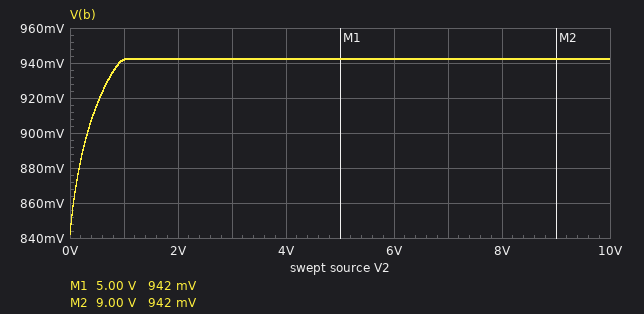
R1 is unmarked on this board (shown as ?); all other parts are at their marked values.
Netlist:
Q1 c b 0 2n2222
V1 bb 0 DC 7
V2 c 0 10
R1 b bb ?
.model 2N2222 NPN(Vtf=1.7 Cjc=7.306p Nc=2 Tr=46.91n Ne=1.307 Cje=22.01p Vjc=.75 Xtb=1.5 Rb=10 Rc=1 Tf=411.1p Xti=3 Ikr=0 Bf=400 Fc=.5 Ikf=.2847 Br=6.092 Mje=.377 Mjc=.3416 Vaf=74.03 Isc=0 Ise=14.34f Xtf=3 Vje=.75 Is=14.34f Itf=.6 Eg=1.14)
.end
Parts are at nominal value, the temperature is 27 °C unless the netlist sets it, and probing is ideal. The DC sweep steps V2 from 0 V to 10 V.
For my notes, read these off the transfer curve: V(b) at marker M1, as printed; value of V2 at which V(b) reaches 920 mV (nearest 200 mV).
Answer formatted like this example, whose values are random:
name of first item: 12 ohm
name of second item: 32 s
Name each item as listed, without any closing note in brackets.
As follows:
V(b) at marker M1, as printed: 942 mV
value of V2 at which V(b) reaches 920 mV: 600 mV
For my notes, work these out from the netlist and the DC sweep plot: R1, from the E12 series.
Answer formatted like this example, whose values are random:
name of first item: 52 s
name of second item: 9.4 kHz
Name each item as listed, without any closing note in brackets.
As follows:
R1, from the E12 series: 680 Ω
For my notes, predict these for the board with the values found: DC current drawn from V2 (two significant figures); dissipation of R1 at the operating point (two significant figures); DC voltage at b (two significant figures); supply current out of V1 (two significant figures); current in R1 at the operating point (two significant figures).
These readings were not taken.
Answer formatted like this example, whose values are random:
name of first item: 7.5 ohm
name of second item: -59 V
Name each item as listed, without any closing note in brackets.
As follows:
DC current drawn from V2: 890 mA
dissipation of R1 at the operating point: 54 mW
DC voltage at b: 940 mV
supply current out of V1: 8.9 mA
current in R1 at the operating point: 8.9 mA
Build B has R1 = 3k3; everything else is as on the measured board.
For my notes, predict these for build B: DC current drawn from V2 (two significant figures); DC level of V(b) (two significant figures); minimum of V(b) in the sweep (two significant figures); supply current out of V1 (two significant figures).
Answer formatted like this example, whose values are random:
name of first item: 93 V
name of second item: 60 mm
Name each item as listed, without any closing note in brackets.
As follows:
DC current drawn from V2: 330 mA
DC level of V(b): 830 mV
minimum of V(b) in the sweep: 730 mV
supply current out of V1: 1.9 mA
